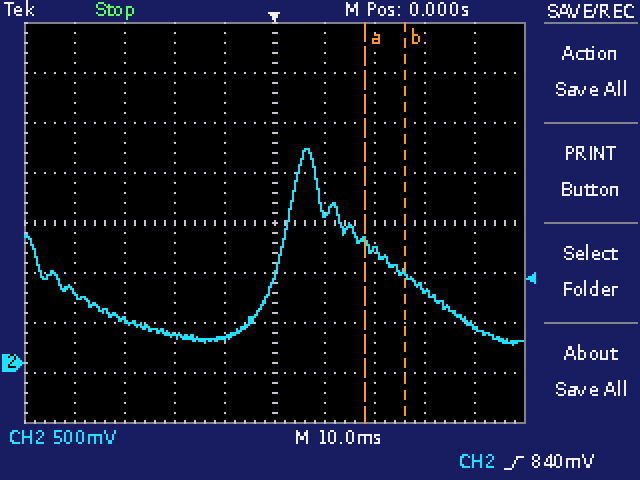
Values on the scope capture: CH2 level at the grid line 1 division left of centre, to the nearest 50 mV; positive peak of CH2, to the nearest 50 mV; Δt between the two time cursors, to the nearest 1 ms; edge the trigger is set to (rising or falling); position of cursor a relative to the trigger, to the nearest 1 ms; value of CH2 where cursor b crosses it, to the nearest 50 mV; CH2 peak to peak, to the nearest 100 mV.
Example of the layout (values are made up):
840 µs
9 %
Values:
250 mV
2.15 V
8 ms
rising
+18 ms
900 mV
2.00 V
